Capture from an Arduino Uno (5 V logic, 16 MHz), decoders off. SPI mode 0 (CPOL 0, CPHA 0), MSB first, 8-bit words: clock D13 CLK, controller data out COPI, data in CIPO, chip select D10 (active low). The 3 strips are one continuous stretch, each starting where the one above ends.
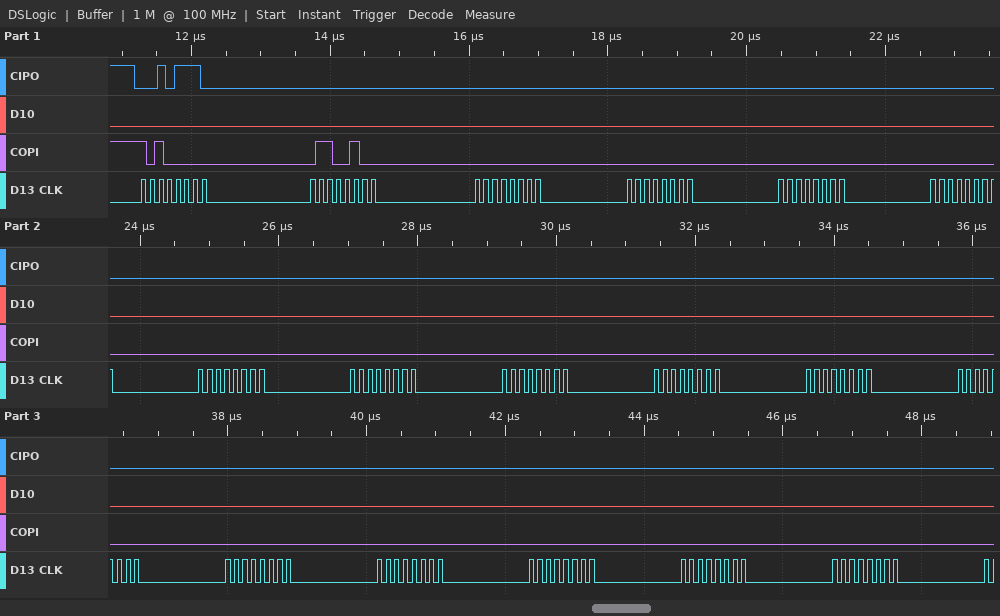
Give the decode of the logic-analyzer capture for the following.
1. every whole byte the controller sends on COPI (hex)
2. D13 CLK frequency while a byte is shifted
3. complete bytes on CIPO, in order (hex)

A0 64 00 00 00 00 00 00 00 00 00 00 00 00 00 00 00
8 MHz
2E 00 00 00 00 00 00 00 00 00 00 00 00 00 00 00 00
